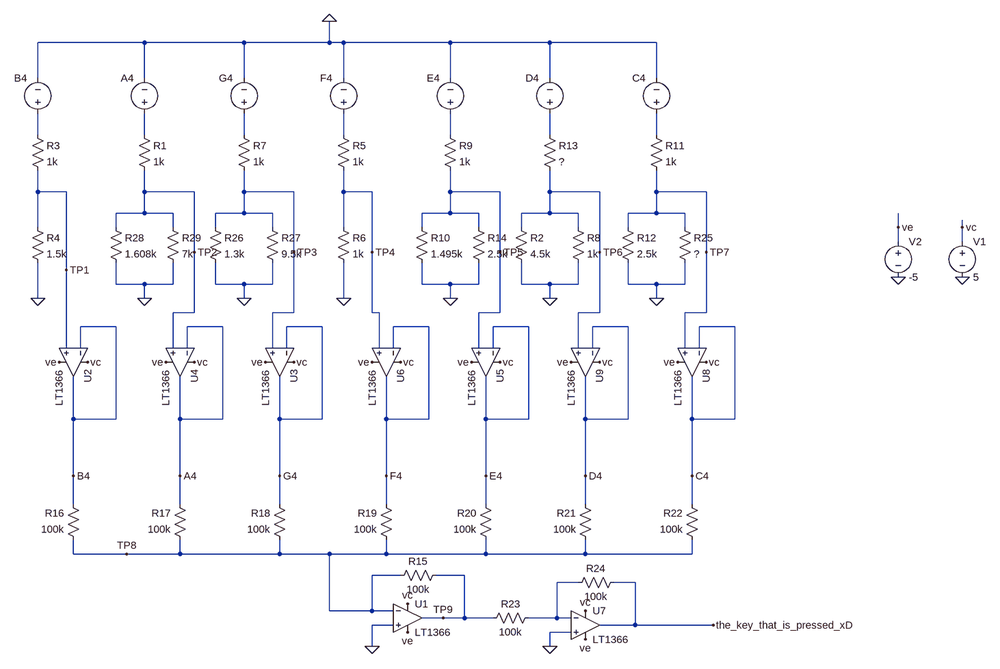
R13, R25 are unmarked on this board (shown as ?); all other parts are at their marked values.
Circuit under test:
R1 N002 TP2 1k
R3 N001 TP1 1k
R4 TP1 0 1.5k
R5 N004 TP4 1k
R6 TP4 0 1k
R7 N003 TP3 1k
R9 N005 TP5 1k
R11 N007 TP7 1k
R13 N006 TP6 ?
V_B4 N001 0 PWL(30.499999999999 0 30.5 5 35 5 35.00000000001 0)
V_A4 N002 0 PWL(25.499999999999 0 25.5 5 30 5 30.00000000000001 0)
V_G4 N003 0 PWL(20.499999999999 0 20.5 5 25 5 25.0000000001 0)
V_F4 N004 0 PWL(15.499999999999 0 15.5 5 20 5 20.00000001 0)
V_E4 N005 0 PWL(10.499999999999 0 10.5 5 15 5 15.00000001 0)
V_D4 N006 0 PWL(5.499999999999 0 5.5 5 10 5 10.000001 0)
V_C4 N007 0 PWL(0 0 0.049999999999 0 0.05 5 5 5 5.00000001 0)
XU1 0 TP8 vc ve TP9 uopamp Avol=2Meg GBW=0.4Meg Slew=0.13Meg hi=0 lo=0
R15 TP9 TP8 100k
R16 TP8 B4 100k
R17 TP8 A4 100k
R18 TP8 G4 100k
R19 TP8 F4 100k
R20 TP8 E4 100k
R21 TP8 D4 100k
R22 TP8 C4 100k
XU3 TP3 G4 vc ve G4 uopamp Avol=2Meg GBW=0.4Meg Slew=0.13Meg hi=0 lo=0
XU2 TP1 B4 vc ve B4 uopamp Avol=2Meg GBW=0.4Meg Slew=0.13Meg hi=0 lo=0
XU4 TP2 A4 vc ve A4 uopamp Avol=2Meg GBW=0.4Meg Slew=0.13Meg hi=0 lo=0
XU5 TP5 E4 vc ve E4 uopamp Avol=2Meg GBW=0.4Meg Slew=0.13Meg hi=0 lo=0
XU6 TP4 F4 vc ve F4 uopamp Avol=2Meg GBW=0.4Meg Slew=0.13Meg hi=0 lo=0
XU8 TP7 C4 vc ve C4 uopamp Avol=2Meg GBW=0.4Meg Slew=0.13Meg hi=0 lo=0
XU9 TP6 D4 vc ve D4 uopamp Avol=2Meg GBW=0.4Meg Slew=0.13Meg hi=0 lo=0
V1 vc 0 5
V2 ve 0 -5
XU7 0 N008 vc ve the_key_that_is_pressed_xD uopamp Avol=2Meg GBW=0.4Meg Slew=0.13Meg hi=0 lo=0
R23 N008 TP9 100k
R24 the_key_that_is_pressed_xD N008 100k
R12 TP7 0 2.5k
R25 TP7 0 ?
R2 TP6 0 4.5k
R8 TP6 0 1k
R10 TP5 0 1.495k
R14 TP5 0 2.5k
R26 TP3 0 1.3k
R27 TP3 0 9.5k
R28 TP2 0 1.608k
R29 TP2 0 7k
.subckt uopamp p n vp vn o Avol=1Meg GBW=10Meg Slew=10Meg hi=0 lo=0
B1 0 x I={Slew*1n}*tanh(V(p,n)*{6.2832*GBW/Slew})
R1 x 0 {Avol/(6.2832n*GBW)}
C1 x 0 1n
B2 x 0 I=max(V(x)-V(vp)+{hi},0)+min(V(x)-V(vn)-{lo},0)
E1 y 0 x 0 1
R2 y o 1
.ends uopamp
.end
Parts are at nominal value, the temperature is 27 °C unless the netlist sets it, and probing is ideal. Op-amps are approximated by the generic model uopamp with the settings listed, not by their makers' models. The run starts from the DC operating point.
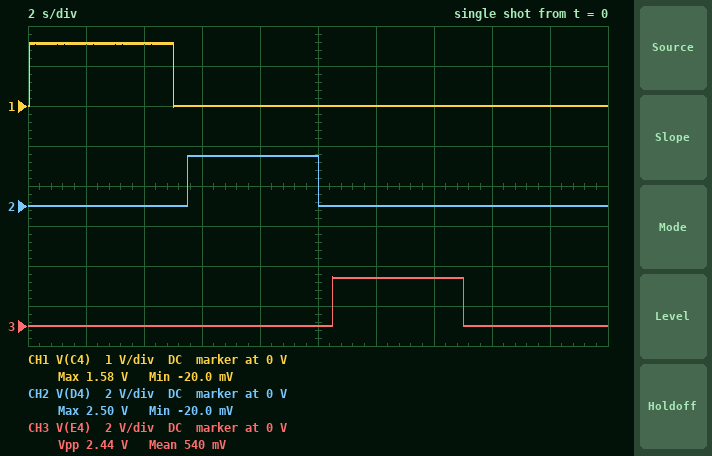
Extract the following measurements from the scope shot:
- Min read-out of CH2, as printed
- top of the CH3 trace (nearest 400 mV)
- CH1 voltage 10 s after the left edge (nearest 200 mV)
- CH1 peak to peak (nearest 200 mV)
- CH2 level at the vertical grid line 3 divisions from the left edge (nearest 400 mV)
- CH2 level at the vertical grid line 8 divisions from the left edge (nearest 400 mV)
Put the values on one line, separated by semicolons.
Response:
-20.0 mV; 2.4 V; 0 V; 1.6 V; 2.4 V; 0 V
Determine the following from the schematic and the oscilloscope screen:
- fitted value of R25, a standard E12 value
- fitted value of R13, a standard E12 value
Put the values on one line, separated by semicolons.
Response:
560 Ω; 820 Ω
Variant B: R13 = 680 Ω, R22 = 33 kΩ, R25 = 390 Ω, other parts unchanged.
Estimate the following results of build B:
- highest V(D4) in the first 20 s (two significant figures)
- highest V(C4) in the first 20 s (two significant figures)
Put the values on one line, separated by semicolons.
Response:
2.7 V; 1.3 V
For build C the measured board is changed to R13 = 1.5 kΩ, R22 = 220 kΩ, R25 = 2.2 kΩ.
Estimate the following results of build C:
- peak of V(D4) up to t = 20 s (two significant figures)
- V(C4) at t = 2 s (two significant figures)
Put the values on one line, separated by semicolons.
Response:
1.8 V; 2.7 V
